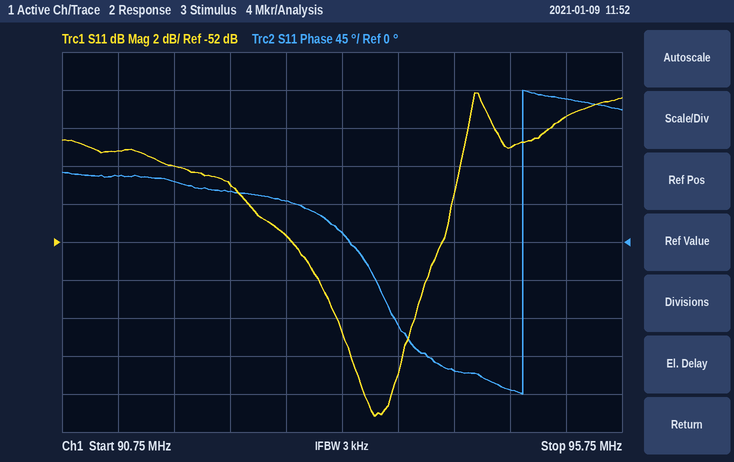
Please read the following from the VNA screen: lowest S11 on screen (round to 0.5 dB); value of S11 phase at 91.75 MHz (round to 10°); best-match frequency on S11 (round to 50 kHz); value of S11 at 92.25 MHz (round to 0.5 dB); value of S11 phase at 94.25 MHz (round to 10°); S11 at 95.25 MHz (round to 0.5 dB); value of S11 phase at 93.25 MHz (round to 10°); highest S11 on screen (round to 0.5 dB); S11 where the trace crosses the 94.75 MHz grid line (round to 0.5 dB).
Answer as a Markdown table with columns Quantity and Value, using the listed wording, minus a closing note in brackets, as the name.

| Quantity | Value |
|---|---|
| lowest S11 on screen | -61.0 dB |
| value of S11 phase at 91.75 MHz | 70° |
| best-match frequency on S11 | 93.55 MHz |
| value of S11 at 92.25 MHz | -49.0 dB |
| value of S11 phase at 94.25 MHz | -150° |
| S11 at 95.25 MHz | -45.5 dB |
| value of S11 phase at 93.25 MHz | 10° |
| highest S11 on screen | -44.0 dB |
| S11 where the trace crosses the 94.75 MHz grid line | -47.0 dB |
